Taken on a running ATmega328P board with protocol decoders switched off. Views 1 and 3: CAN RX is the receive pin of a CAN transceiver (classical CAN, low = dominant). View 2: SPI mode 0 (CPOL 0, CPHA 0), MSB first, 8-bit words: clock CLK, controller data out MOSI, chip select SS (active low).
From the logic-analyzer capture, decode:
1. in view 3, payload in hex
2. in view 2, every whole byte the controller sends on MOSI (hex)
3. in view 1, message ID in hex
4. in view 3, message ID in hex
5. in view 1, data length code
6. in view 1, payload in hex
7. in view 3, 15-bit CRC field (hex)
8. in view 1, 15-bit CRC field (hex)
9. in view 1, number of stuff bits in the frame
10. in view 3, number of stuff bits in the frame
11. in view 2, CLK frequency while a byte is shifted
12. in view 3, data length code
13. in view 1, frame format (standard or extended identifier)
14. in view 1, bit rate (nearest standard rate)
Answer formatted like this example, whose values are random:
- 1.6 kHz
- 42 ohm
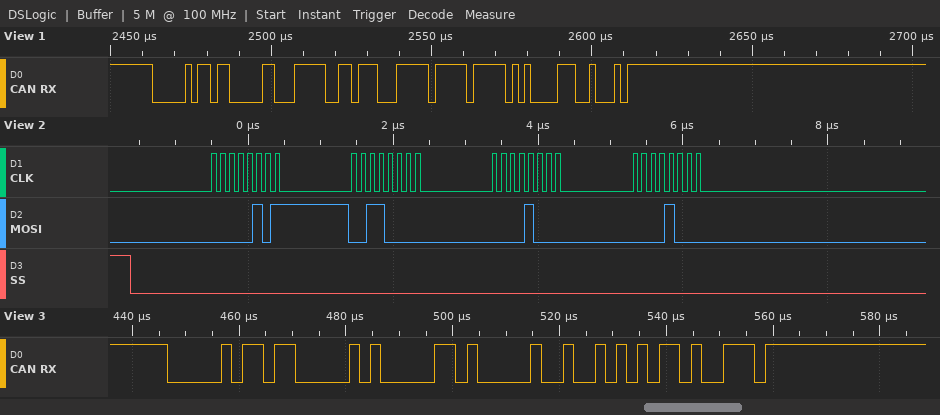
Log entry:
- 0A 02
- 05 30 08 08
- 0x036
- 0x036
- 4
- 7D B8 FF FF
- 0x2AD3
- 0x21C8
- 6
- 4
- 8 MHz
- 2
- standard
- 500 kbit/s
